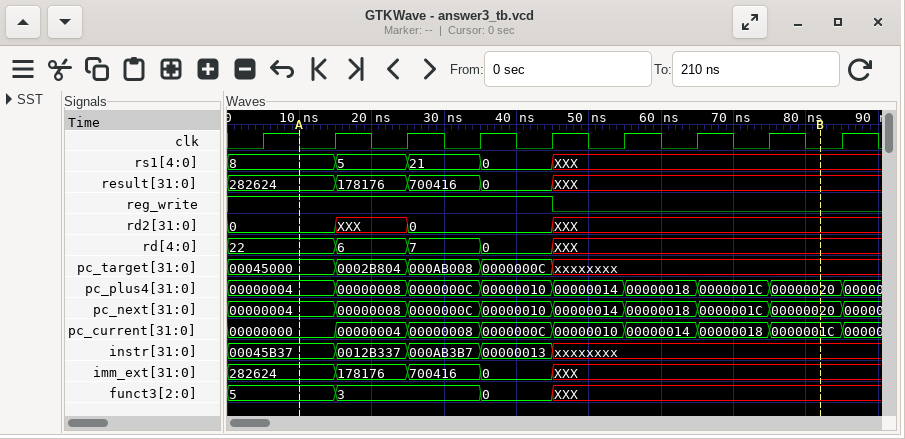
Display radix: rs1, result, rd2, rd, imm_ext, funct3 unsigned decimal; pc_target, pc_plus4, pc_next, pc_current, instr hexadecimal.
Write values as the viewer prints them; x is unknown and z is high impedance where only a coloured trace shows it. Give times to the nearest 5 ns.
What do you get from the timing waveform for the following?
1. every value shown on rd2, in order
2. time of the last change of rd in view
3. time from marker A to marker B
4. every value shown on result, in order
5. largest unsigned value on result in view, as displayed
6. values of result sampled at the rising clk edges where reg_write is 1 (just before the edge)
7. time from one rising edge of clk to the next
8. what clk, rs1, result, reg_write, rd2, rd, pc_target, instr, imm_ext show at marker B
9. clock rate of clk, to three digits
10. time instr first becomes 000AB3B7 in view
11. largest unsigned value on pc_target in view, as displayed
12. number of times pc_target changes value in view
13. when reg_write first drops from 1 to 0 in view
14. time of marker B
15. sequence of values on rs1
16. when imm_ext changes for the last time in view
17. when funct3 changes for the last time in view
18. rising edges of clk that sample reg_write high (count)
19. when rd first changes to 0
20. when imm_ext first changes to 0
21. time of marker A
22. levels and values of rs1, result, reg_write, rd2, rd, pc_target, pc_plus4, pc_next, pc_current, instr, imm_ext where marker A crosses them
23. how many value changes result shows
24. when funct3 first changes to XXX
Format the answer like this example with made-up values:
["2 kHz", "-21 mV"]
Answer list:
["0, XXX, 0, XXX", "45 ns", "70 ns", "282624, 178176, 700416, 0, XXX", "700416", "282624, 282624, 178176, 700416, 0", "10 ns", "clk=0, rs1=XXX, result=XXX, reg_write=0, rd2=XXX, rd=XXX, pc_target=xxxxxxxx, instr=xxxxxxxx, imm_ext=XXX", "100 MHz", "25 ns", "000AB008", "4", "45 ns", "80 ns", "8, 5, 21, 0, XXX", "45 ns", "45 ns", "5", "35 ns", "35 ns", "10 ns", "rs1=8, result=282624, reg_write=1, rd2=0, rd=22, pc_target=00045000, pc_plus4=00000004, pc_next=00000004, pc_current=00000000, instr=00045B37, imm_ext=282624", "4", "45 ns"]
